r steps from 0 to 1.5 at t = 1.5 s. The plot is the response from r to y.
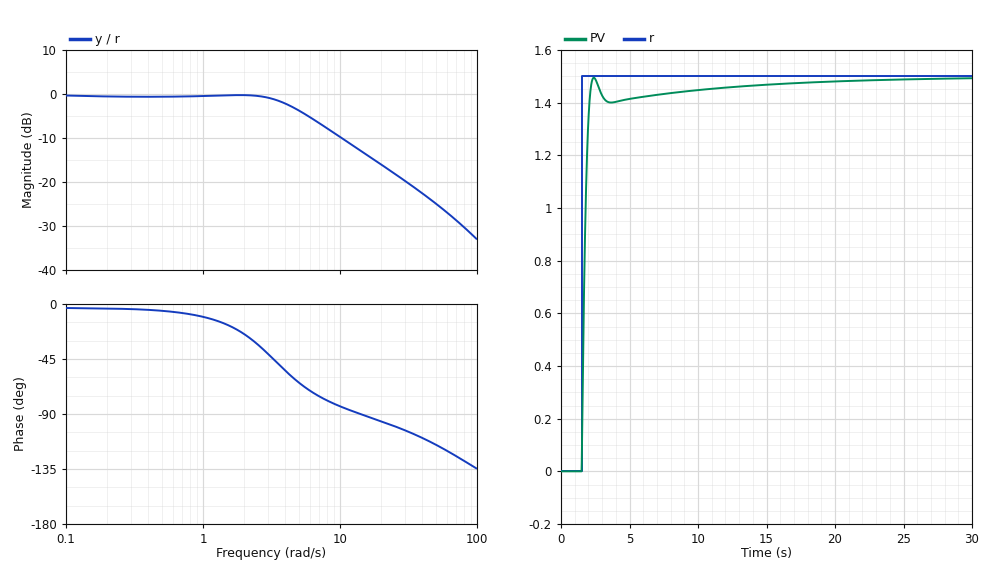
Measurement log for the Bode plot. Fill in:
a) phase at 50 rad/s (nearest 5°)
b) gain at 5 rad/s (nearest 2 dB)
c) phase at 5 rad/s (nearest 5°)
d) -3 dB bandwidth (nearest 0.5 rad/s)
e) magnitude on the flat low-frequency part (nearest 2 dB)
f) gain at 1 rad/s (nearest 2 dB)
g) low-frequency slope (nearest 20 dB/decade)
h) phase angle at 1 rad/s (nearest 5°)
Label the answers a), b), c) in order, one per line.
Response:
a) -115°
b) -4 dB
c) -65°
d) 5.0 rad/s
e) 0 dB
f) 0 dB
g) 0 dB/decade
h) -10°
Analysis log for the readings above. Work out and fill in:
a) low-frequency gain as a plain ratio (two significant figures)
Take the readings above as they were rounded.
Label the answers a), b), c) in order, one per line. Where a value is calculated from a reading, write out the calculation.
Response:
a) 10^(0 / 20) = 1.0
